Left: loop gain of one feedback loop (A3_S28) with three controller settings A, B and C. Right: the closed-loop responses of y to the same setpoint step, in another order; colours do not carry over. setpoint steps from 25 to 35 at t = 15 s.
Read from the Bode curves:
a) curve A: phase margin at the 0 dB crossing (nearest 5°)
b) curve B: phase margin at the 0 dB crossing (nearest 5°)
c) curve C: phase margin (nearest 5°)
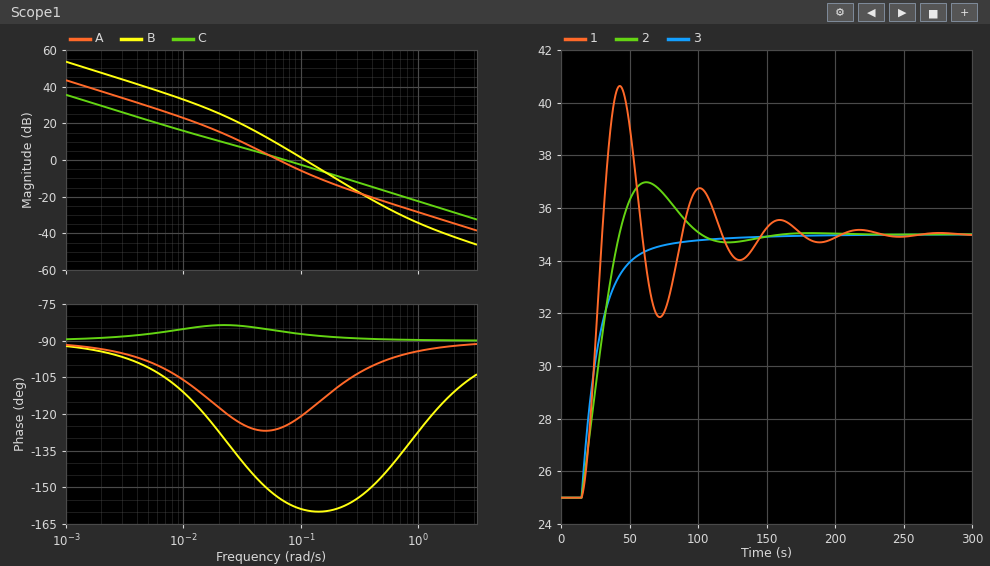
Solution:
55°
20°
95°
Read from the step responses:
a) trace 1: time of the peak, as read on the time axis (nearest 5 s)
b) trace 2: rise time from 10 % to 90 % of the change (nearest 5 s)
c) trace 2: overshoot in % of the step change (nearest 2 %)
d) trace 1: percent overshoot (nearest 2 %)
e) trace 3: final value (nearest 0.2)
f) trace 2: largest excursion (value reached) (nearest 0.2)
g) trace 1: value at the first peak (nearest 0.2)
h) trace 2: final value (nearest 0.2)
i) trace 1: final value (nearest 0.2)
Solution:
45 s
20 s
20 %
56 %
35.0
37.0
40.6
35.0
35.0
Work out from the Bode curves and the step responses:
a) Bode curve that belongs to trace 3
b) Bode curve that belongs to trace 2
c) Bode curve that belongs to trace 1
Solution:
C
A
B
